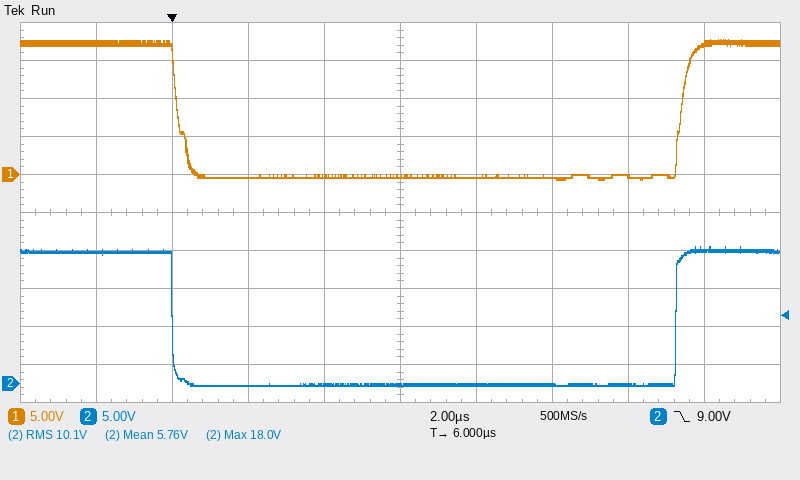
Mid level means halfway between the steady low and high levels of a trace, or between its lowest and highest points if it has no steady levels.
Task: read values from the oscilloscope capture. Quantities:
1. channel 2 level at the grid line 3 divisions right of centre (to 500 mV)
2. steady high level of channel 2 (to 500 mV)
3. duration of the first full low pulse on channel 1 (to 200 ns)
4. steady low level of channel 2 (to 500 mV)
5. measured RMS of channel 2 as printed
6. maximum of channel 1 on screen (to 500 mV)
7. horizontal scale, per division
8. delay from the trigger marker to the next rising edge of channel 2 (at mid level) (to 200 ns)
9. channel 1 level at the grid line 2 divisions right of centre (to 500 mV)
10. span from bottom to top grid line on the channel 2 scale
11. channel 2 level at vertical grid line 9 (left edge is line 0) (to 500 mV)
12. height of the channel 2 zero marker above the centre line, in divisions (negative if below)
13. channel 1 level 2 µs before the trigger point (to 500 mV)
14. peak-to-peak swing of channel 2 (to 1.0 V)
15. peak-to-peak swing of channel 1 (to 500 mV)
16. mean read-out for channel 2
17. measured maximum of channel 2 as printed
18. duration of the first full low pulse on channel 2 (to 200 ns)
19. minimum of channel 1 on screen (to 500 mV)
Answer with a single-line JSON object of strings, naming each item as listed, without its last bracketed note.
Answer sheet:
{"channel 2 level at the grid line 3 divisions right of centre": "0.0 V", "steady high level of channel 2": "17.5 V", "duration of the first full low pulse on channel 1": "13.2 µs", "steady low level of channel 2": "0.0 V", "measured RMS of channel 2 as printed": "10.1 V", "maximum of channel 1 on screen": "18.0 V", "horizontal scale, per division": "2 µs", "delay from the trigger marker to the next rising edge of channel 2 (at mid level)": "13.2 µs", "channel 1 level at the grid line 2 divisions right of centre": "-500 mV", "span from bottom to top grid line on the channel 2 scale": "50 V", "channel 2 level at vertical grid line 9 (left edge is line 0)": "17.5 V", "height of the channel 2 zero marker above the centre line, in divisions": "-4.5 div", "channel 1 level 2 µs before the trigger point": "17.5 V", "peak-to-peak swing of channel 2": "18.0 V", "peak-to-peak swing of channel 1": "18.5 V", "mean read-out for channel 2": "5.76 V", "measured maximum of channel 2 as printed": "18.0 V", "duration of the first full low pulse on channel 2": "13.2 µs", "minimum of channel 1 on screen": "-500 mV"}
